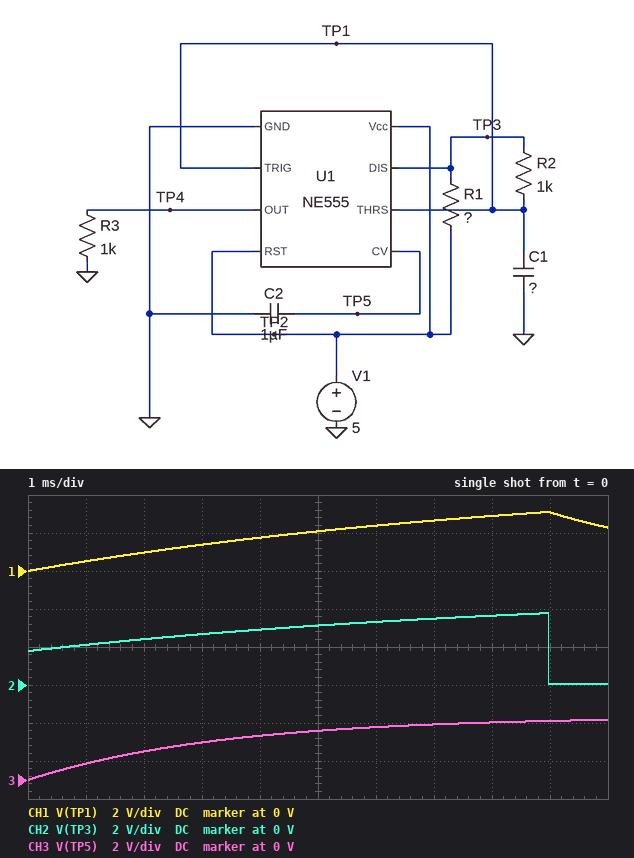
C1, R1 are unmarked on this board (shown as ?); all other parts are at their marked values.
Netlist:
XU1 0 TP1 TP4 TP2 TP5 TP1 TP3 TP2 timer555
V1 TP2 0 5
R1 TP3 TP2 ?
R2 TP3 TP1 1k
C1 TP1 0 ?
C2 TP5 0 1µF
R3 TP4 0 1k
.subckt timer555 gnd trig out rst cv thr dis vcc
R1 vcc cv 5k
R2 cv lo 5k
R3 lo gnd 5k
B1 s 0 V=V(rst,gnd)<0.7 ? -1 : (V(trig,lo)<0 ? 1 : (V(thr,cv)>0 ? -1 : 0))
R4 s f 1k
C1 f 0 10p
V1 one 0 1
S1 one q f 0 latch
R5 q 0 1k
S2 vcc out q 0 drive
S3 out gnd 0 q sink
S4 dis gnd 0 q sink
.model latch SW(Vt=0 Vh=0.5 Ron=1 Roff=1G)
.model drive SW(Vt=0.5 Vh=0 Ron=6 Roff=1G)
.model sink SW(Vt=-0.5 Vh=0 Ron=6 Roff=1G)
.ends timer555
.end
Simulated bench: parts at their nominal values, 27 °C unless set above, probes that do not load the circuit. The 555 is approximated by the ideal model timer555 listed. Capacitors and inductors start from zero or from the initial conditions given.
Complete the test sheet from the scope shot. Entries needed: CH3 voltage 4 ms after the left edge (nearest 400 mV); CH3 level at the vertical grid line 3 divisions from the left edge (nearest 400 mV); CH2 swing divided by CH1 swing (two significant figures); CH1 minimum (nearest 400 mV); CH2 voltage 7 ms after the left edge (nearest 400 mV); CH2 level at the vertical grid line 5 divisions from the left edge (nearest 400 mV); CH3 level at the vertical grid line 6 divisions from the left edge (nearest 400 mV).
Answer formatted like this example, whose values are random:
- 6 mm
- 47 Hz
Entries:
- 2.4 V
- 2.0 V
- 1.2
- 0 V
- 3.6 V
- 3.2 V
- 2.8 V
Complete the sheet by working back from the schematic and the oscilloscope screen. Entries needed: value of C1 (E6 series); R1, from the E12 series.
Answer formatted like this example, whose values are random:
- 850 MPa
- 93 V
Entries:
- 3.3 µF
- 1.8 kΩ
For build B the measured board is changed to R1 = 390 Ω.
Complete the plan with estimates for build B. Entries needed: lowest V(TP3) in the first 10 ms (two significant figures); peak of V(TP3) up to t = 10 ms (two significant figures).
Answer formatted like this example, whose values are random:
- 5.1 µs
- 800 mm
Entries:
- 75 mV
- 4.4 V
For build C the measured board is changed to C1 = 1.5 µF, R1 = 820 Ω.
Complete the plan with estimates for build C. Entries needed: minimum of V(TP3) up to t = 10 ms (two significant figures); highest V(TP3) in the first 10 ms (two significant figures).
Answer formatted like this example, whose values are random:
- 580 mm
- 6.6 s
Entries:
- 36 mV
- 4.1 V
